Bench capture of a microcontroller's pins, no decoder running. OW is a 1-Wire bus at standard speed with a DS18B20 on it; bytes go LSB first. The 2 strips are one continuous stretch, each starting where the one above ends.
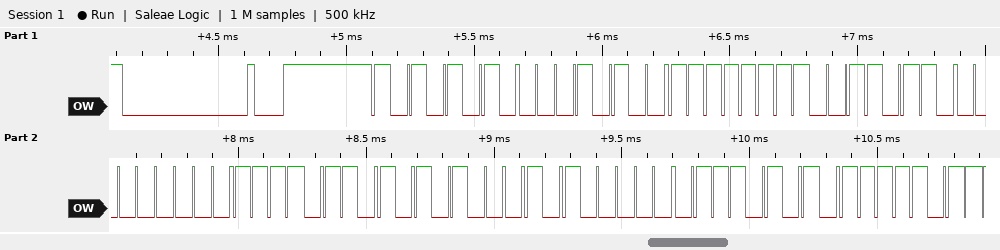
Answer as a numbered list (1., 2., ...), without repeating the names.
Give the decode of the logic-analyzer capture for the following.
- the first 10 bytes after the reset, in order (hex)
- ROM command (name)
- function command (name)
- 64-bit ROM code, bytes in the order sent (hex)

1. 55 28 FF 6C 00 6F 15 05 AE BE
2. Match ROM
3. Read Scratchpad
4. 28 FF 6C 00 6F 15 05 AE
